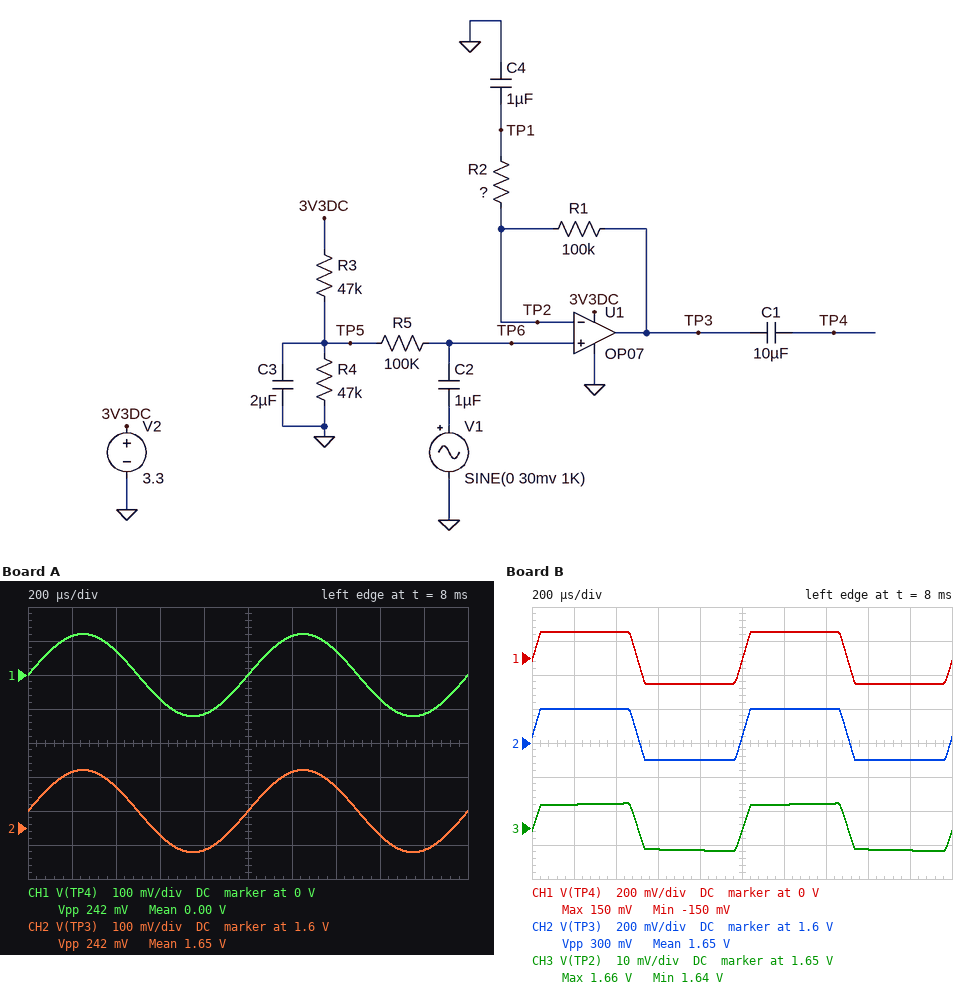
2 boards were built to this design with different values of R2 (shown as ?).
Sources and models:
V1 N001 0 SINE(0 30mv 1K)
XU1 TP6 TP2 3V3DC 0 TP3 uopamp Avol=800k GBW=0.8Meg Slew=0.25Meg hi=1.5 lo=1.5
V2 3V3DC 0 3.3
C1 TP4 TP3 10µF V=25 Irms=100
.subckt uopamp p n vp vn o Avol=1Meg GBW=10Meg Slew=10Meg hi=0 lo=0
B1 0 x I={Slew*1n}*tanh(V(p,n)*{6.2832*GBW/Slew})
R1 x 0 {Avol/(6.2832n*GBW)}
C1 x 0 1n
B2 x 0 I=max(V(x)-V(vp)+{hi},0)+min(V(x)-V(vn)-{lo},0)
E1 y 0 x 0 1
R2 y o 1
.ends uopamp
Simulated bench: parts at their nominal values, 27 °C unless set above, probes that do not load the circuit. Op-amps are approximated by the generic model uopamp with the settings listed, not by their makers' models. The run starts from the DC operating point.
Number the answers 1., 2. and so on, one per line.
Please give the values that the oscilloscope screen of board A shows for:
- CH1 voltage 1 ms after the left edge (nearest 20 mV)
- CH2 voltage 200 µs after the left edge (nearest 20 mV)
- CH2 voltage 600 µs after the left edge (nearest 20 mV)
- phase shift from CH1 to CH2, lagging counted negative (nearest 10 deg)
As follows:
1. 0 V
2. 1.76 V
3. 1.58 V
4. 0 deg
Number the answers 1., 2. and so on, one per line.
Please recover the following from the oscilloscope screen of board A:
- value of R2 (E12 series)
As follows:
1. 33 kΩ
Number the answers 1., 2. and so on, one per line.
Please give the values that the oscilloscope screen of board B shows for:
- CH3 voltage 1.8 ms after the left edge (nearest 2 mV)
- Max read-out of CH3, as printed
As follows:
1. 1.644 V
2. 1.66 V
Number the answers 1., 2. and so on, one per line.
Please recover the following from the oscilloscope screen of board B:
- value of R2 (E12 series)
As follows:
1. 4.7 kΩ
